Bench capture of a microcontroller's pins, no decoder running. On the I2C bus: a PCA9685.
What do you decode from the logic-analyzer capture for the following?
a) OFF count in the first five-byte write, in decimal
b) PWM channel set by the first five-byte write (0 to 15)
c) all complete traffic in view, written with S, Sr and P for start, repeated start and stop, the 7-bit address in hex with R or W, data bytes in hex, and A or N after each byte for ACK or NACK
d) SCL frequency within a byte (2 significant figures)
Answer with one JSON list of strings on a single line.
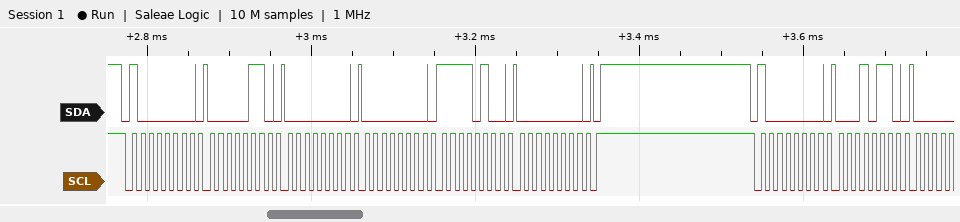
["244", "0", "S 40W A 06 A 00 A 00 A F4 A 00 A P S 40W A 16 A", "100 kHz"]
